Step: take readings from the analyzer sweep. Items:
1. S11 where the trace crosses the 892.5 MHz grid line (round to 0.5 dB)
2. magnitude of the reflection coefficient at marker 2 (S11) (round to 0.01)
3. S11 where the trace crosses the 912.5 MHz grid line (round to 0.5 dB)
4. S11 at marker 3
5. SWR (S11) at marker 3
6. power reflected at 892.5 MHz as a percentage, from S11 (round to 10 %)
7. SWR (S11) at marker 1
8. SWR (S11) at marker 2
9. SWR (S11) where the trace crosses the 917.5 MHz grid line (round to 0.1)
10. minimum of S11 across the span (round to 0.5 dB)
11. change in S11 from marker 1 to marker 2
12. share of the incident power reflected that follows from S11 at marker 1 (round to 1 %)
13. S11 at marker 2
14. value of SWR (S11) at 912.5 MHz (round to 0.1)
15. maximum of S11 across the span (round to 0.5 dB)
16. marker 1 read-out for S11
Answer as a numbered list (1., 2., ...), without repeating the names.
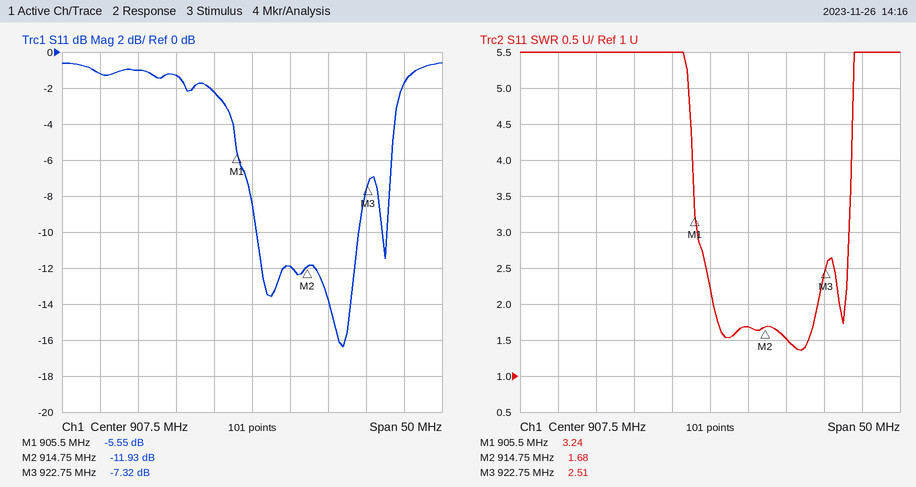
1. -1.0 dB
2. 0.25
3. -12.0 dB
4. -7.32 dB
5. 2.51
6. 80 %
7. 3.24
8. 1.68
9. 1.5
10. -16.5 dB
11. -6.38 dB
12. 28 %
13. -11.93 dB
14. 1.7
15. -0.5 dB
16. -5.55 dB
